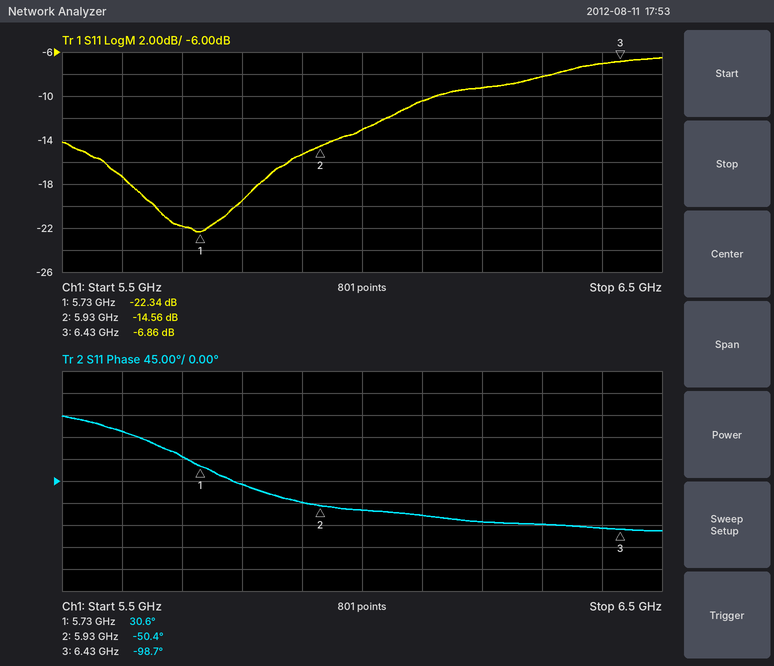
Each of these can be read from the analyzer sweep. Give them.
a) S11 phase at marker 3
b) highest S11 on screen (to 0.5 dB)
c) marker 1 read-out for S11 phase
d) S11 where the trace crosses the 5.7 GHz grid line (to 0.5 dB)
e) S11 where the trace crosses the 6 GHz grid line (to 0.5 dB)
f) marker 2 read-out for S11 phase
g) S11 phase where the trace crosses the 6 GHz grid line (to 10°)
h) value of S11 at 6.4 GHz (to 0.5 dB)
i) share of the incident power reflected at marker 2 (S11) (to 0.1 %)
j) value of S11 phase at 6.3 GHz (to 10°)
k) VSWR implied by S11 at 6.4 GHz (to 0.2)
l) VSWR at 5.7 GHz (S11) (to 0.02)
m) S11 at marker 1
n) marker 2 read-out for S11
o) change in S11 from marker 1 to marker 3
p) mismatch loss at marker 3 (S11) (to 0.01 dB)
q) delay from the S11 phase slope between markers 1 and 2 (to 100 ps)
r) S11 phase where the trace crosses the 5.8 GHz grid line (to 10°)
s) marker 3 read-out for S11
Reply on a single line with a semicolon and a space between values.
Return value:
-98.7°; -6.5 dB; 30.6°; -22.0 dB; -13.0 dB; -50.4°; -60°; -7.0 dB; 3.5 %; -90°; 2.6; 1.18; -22.34 dB; -14.56 dB; 15.48 dB; 1.00 dB; 1.1 ns; -10°; -6.86 dB
